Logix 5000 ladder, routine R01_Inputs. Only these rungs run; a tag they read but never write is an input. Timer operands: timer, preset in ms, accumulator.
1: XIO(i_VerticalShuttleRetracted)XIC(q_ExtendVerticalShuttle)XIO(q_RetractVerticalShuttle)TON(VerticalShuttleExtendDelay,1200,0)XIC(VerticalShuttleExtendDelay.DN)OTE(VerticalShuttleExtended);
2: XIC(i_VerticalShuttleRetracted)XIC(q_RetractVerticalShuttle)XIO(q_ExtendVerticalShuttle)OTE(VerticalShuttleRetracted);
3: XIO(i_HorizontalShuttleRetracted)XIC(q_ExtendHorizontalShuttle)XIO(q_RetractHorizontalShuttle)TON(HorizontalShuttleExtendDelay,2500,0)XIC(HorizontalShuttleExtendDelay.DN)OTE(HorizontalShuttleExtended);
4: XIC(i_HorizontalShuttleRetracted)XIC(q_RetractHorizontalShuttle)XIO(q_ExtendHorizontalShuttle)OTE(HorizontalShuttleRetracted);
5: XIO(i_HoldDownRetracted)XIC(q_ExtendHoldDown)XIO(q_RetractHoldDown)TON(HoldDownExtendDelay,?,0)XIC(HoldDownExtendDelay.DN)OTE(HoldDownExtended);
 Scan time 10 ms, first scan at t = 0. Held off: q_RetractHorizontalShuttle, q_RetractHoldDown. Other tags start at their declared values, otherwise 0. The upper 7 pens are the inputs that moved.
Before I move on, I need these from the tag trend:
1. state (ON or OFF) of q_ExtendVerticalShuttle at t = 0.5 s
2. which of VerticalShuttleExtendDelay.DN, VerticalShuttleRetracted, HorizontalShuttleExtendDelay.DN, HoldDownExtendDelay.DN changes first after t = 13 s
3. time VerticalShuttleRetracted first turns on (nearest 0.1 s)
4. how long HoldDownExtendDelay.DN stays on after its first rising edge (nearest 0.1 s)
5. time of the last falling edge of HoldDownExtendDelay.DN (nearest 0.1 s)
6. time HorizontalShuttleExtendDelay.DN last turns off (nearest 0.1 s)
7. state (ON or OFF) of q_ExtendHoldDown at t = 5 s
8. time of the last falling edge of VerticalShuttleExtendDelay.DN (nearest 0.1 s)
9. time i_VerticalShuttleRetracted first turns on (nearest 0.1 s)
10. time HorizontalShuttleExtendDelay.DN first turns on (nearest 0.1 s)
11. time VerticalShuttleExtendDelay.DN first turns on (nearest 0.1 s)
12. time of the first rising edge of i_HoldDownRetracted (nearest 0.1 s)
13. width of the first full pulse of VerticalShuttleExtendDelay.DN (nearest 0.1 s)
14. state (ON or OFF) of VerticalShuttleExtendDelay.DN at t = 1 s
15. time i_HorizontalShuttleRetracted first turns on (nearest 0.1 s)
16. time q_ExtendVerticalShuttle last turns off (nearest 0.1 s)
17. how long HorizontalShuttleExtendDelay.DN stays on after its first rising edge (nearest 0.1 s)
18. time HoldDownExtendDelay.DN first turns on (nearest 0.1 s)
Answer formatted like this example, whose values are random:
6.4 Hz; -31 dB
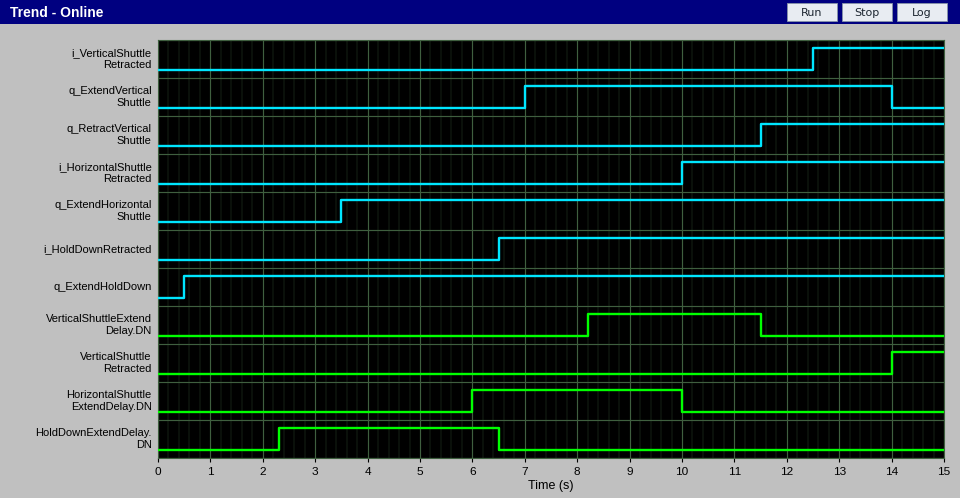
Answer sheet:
OFF; VerticalShuttleRetracted; 14.0 s; 4.2 s; 6.5 s; 10.0 s; ON; 11.5 s; 12.5 s; 6.0 s; 8.2 s; 6.5 s; 3.3 s; OFF; 10.0 s; 14.0 s; 4.0 s; 2.3 s
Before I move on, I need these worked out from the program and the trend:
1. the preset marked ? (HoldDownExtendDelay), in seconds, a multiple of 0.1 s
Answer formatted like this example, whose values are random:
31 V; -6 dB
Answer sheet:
1.8 s
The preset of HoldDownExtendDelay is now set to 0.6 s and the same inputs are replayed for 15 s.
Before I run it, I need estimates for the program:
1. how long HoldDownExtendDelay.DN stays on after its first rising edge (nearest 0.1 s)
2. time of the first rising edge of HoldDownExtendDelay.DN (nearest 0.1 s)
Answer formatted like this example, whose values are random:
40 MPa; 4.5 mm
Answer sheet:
5.4 s; 1.1 s
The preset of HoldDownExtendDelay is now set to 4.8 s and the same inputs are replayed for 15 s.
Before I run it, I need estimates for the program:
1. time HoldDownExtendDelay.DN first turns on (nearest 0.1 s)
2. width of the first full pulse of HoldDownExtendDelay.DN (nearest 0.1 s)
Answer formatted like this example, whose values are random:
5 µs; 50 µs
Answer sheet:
5.3 s; 1.2 s
